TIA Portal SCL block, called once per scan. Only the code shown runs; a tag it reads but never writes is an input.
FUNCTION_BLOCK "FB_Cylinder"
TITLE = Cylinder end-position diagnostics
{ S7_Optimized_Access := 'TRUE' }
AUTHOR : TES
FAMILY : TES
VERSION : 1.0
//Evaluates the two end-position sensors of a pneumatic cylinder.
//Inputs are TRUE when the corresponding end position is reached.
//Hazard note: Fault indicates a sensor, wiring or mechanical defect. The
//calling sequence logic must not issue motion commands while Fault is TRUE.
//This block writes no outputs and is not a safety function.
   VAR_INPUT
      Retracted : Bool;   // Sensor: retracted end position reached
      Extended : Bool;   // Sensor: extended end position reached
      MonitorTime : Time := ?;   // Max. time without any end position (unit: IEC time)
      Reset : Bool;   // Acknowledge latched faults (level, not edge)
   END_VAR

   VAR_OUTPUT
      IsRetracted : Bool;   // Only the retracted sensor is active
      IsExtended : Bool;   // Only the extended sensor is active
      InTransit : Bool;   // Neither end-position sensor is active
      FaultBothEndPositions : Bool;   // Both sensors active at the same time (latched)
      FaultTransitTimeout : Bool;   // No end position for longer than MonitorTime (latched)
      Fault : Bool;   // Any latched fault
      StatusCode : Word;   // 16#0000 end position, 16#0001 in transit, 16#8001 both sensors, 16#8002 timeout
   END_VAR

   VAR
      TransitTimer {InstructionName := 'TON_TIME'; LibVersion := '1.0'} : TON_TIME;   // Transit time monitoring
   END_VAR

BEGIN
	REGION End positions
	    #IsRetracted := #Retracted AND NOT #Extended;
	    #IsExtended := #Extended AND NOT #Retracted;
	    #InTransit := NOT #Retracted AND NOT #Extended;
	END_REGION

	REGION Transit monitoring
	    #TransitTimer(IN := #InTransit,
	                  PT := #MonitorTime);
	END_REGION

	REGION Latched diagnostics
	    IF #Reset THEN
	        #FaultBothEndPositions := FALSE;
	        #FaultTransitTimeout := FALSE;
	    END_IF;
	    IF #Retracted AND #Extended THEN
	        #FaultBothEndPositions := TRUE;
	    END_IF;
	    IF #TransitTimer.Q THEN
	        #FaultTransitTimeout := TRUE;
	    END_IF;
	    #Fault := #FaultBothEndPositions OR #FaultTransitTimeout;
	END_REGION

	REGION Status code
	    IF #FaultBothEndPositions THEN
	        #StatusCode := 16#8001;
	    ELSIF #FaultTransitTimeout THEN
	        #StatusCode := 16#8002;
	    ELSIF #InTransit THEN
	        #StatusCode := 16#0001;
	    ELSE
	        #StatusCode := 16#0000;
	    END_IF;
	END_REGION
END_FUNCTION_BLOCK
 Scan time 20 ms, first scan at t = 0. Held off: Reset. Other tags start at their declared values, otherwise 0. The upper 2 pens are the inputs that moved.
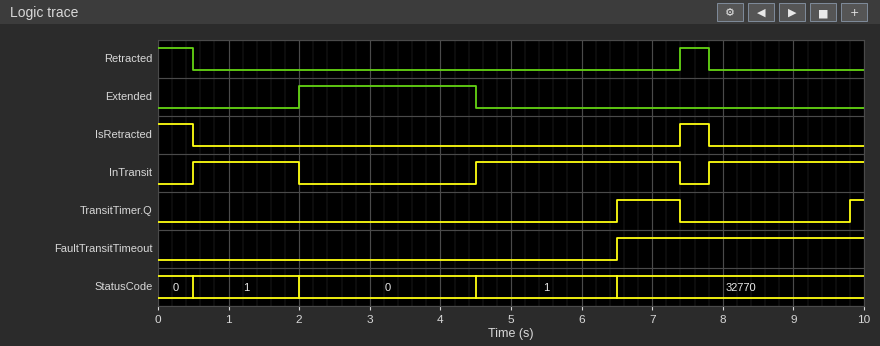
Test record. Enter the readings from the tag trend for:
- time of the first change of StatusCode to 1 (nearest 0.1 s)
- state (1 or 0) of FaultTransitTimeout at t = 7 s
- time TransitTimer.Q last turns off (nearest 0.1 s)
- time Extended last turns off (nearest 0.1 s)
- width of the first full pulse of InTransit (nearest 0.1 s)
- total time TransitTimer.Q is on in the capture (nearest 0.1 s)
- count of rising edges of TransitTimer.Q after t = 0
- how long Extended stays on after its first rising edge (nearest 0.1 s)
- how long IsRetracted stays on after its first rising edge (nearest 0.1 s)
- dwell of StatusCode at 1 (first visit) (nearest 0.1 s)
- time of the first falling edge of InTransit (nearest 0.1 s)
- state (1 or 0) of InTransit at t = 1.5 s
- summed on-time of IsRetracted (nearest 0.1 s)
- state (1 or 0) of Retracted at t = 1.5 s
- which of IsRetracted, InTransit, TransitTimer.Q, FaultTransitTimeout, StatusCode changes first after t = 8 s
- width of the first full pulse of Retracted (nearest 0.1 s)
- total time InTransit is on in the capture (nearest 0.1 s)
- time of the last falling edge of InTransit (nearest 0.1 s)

0.5 s
1
7.4 s
4.5 s
1.5 s
1.1 s
2
2.5 s
0.4 s
1.5 s
2.0 s
1
0.9 s
0
TransitTimer.Q
0.4 s
6.6 s
7.4 s
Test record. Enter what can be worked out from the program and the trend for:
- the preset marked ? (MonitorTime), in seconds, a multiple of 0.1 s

2.0 s
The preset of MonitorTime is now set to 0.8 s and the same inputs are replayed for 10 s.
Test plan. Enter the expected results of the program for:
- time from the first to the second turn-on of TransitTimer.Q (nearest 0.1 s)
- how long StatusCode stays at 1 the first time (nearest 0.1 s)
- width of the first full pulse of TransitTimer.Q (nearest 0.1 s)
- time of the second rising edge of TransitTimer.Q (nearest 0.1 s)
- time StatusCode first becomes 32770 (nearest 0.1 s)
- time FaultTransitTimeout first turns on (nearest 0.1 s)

4.0 s
0.8 s
0.7 s
5.3 s
1.3 s
1.3 s
